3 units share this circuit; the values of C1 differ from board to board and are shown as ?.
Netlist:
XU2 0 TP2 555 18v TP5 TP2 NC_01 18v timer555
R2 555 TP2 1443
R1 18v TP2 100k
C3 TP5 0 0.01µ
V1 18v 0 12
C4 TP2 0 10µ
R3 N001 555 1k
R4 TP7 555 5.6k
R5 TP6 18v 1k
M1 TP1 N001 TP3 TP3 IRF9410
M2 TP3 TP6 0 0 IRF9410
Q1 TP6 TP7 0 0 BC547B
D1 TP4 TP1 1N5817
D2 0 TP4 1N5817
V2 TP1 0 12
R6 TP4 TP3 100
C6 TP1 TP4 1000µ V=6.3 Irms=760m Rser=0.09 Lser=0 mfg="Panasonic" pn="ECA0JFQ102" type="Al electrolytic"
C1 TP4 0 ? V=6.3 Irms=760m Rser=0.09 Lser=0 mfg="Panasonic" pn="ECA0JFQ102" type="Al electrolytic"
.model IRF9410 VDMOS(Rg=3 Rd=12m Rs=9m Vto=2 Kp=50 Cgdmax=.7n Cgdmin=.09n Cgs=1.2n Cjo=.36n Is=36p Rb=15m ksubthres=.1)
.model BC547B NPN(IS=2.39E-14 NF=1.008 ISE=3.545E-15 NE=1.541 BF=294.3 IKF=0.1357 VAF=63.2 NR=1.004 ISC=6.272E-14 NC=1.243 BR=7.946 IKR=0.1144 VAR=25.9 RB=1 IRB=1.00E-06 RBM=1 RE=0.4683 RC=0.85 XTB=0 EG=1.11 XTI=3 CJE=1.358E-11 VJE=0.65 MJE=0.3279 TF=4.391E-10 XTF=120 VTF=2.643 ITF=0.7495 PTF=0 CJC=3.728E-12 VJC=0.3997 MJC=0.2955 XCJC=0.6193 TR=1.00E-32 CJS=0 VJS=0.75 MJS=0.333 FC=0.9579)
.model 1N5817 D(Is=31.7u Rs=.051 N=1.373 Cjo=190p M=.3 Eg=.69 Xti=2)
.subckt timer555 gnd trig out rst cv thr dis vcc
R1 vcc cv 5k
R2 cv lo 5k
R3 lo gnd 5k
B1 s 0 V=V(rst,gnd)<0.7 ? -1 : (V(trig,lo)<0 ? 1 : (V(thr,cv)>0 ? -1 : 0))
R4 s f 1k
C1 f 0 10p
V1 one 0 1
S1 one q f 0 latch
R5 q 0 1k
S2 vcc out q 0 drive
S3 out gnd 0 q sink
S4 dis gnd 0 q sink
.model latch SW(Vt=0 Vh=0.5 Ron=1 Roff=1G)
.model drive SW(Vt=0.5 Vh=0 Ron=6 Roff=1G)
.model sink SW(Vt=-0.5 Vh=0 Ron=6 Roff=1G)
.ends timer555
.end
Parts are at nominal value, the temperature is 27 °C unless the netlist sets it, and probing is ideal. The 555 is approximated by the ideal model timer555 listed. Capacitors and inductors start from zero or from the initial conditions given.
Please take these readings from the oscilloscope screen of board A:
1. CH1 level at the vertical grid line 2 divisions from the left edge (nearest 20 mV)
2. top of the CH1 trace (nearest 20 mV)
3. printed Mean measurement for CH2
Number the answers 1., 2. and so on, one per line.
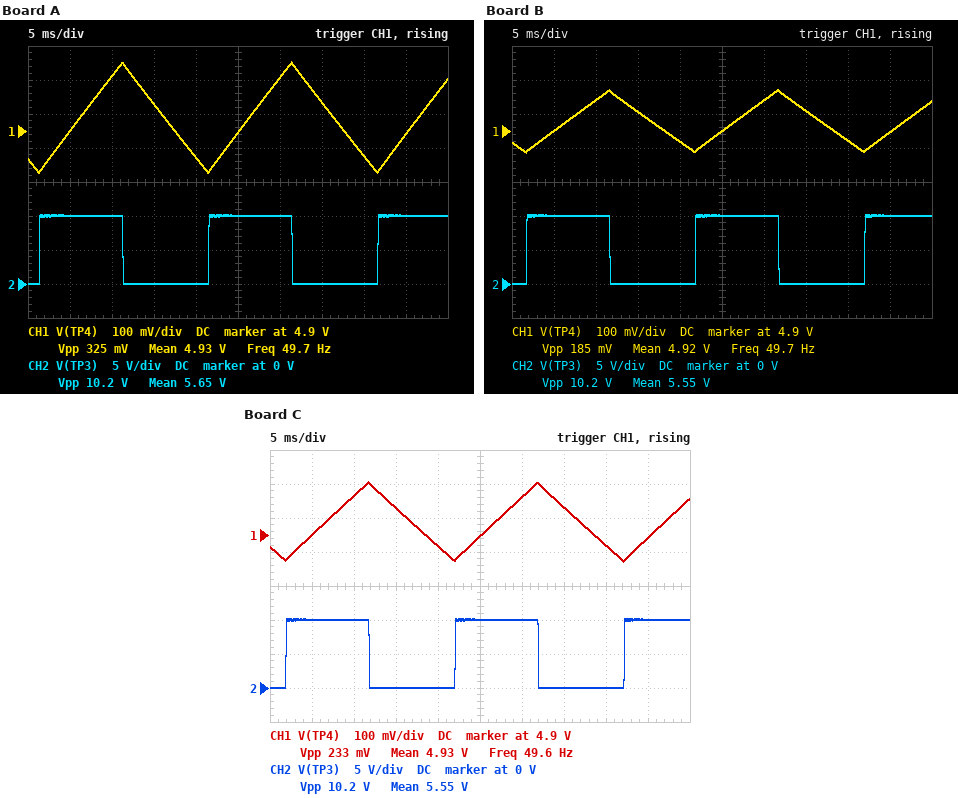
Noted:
1. 5.06 V
2. 5.10 V
3. 5.65 V
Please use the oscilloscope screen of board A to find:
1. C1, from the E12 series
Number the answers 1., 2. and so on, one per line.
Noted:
1. 560 µF
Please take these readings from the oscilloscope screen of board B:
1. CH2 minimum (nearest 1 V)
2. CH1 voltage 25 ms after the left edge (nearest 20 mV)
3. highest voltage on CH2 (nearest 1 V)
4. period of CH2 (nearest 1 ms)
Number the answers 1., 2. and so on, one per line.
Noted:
1. 0 V
2. 4.90 V
3. 10 V
4. 20 ms
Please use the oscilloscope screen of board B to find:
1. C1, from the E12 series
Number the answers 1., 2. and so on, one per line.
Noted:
1. 1.8 mF
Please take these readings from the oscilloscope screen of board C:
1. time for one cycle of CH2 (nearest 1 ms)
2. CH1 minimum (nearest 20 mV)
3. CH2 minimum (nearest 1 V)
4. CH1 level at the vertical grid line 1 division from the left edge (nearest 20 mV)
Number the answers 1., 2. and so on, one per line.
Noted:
1. 20 ms
2. 4.82 V
3. 0 V
4. 4.90 V
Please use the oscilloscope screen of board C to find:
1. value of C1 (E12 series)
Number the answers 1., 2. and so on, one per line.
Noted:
1. 1.2 mF
